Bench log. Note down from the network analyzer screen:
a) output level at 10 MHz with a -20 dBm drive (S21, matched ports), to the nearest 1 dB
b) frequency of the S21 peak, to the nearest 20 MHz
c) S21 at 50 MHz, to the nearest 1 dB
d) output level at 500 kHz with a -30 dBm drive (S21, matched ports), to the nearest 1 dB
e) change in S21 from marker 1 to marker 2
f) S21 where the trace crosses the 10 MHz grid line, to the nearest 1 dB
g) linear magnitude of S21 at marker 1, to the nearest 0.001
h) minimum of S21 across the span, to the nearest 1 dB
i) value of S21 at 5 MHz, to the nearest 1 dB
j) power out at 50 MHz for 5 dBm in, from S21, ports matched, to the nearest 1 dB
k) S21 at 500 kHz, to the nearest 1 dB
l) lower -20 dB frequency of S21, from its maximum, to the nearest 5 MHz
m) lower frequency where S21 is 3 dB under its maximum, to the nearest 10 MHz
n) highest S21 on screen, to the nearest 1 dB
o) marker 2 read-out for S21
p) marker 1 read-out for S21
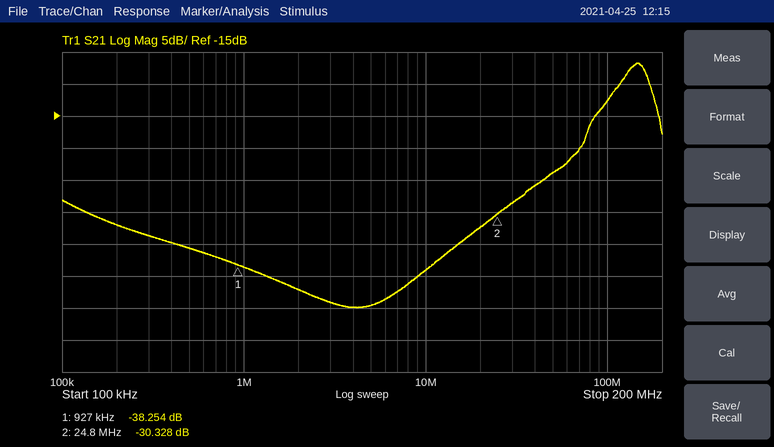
-59 dBm
140 MHz
-24 dB
-66 dBm
7.926 dB
-39 dB
0.012
-45 dB
-45 dB
-19 dBm
-36 dB
35 MHz
120 MHz
-7 dB
-30.328 dB
-38.254 dB
